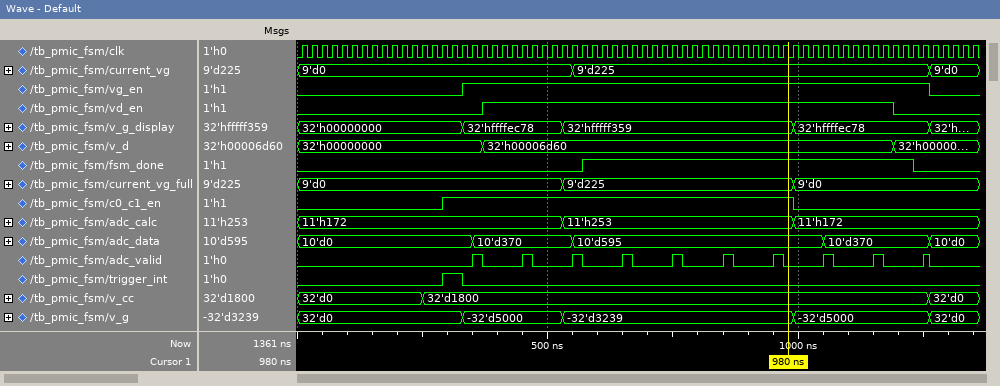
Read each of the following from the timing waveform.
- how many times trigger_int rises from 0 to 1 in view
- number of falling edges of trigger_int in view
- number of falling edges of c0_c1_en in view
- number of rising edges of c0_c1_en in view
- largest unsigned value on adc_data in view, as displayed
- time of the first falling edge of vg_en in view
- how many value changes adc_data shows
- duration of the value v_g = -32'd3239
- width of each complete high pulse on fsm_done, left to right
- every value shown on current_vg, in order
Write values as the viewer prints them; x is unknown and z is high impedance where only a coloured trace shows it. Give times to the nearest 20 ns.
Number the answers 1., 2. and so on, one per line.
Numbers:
1. 1
2. 1
3. 1
4. 1
5. 10'd595
6. 1260 ns
7. 4
8. 460 ns
9. 660 ns
10. 9'd0, 9'd225, 9'd0
